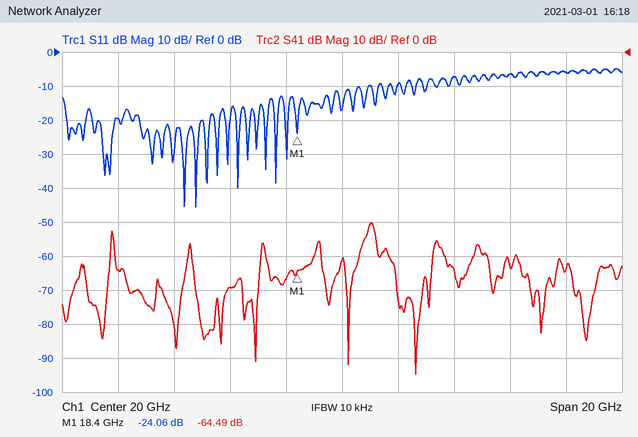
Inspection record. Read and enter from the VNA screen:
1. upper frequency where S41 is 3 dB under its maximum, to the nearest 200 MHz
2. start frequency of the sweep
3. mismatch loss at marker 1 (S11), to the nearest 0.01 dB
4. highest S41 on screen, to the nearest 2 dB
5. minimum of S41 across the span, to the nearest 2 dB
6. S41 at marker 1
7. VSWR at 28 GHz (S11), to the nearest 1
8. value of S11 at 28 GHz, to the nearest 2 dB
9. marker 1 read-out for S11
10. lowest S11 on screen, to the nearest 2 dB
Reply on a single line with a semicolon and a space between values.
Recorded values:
21.2 GHz; 10 GHz; 0.02 dB; -50 dB; -94 dB; -64.49 dB; 3; -6 dB; -24.06 dB; -46 dB
